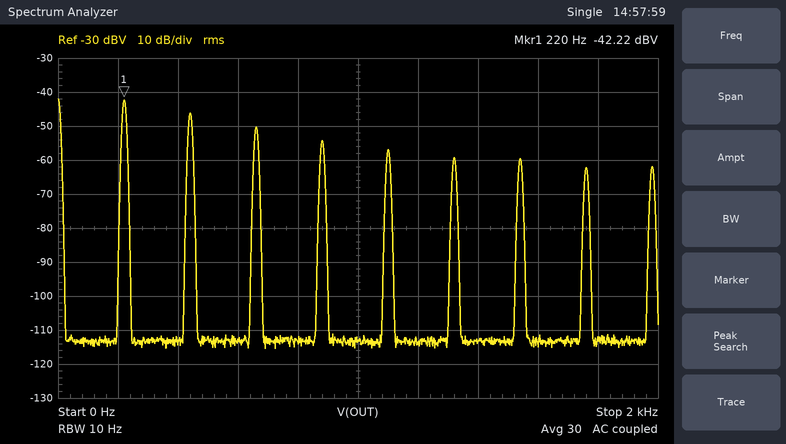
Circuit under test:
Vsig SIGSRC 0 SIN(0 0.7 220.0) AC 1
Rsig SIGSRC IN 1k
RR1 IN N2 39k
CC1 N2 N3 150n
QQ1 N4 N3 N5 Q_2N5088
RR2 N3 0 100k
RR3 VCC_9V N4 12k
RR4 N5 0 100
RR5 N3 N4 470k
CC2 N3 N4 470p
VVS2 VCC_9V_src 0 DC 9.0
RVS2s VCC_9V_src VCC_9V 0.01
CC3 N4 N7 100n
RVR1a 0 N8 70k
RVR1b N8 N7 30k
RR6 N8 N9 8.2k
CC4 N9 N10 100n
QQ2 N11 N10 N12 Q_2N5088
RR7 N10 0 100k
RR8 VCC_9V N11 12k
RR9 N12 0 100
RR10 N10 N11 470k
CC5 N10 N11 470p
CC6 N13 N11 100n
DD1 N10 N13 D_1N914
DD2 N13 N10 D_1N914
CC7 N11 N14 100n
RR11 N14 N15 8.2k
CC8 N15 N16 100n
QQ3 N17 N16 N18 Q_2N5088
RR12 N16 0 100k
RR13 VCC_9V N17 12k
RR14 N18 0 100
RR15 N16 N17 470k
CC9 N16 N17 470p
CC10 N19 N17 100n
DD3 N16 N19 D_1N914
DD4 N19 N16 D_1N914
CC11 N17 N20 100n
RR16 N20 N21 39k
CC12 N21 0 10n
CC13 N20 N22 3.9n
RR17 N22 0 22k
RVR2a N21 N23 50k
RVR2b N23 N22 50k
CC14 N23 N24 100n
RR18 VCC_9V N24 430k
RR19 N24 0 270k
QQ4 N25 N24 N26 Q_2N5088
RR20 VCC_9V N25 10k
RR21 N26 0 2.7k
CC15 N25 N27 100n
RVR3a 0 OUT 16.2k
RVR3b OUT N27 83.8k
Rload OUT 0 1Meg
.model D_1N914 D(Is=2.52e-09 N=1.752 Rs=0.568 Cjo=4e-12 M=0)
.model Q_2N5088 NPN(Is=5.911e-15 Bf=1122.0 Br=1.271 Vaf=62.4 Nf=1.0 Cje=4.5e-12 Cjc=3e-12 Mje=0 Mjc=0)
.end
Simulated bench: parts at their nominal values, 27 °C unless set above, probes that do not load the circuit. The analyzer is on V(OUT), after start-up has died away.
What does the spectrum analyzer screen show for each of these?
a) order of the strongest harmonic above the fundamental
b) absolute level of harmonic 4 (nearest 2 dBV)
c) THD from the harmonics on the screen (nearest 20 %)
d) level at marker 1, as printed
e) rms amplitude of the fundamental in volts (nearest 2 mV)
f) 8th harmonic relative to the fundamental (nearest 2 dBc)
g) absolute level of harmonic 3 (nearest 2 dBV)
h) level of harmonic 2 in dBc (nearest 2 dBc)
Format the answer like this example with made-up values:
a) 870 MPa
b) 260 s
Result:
a) 2
b) -54 dBV
c) 80 %
d) -42.22 dBV
e) 8 mV
f) -20 dBc
g) -50 dBV
h) -4 dBc
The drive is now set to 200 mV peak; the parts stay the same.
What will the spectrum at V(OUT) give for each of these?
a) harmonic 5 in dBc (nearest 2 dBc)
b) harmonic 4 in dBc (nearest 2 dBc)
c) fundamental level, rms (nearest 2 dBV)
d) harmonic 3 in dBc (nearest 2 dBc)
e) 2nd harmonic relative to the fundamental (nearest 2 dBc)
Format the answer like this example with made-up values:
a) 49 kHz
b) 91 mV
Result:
a) -22 dBc
b) -20 dBc
c) -52 dBV
d) -20 dBc
e) -8 dBc
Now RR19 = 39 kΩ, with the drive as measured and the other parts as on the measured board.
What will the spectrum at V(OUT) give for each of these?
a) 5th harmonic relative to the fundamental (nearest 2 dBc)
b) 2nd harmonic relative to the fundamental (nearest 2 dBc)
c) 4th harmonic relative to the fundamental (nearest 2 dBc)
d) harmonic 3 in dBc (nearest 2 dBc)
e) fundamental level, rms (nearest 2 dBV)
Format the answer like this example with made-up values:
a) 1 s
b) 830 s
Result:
a) -22 dBc
b) -32 dBc
c) -34 dBc
d) -16 dBc
e) -28 dBV
